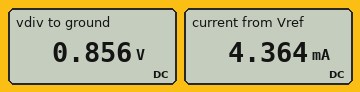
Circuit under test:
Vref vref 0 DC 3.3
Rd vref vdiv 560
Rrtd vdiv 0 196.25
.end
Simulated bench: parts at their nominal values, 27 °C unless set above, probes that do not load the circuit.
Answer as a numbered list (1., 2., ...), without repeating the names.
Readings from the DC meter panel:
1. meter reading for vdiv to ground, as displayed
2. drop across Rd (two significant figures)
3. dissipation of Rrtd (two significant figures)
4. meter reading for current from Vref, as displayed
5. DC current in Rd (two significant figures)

1. 0.856 V
2. 2.4 V
3. 3.7 mW
4. 4.364 mA
5. 4.4 mA
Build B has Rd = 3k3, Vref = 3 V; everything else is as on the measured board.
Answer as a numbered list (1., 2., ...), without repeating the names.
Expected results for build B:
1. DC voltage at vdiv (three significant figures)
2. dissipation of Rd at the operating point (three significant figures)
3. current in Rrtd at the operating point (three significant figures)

1. 168 mV
2. 2.43 mW
3. 858 µA
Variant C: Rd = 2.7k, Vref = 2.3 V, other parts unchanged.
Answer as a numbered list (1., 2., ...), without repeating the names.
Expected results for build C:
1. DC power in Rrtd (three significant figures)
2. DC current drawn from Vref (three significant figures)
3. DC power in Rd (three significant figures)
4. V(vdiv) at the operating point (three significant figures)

1. 124 µW
2. 794 µA
3. 1.70 mW
4. 156 mV
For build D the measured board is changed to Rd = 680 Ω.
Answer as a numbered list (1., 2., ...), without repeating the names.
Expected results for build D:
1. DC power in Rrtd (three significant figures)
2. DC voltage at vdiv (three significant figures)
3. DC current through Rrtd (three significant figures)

1. 2.78 mW
2. 739 mV
3. 3.77 mA
